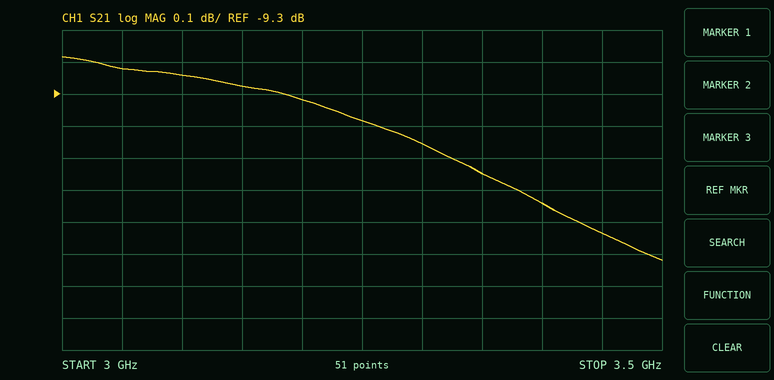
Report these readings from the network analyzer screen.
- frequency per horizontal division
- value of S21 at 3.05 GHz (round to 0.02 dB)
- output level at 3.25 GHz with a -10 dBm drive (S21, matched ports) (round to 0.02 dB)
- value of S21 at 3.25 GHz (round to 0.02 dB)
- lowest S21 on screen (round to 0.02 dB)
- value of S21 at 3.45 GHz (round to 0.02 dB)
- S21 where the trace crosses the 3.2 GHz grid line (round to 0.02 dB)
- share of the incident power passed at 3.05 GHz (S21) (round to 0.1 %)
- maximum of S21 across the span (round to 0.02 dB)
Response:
50 MHz
-9.22 dB
-19.38 dBm
-9.38 dB
-9.82 dB
-9.74 dB
-9.32 dB
12.0 %
-9.18 dB
